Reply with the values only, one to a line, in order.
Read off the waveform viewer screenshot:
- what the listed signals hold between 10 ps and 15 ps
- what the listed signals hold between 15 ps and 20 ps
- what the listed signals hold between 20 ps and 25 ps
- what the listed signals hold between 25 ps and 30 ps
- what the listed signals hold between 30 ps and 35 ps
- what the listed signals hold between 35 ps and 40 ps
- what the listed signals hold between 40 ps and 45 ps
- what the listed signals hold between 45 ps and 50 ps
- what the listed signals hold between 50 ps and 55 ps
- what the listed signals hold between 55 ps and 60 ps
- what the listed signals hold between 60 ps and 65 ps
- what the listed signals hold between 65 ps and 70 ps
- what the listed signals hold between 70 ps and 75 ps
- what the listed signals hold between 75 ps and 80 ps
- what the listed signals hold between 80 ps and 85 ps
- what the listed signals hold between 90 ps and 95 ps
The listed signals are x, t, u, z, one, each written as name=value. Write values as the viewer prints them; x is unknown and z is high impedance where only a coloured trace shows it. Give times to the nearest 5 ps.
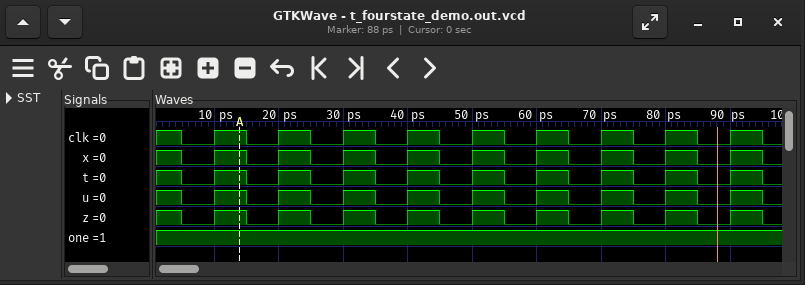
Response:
x=1, t=1, u=1, z=1, one=1
x=0, t=0, u=0, z=0, one=1
x=1, t=1, u=1, z=1, one=1
x=0, t=0, u=0, z=0, one=1
x=1, t=1, u=1, z=1, one=1
x=0, t=0, u=0, z=0, one=1
x=1, t=1, u=1, z=1, one=1
x=0, t=0, u=0, z=0, one=1
x=1, t=1, u=1, z=1, one=1
x=0, t=0, u=0, z=0, one=1
x=1, t=1, u=1, z=1, one=1
x=0, t=0, u=0, z=0, one=1
x=1, t=1, u=1, z=1, one=1
x=0, t=0, u=0, z=0, one=1
x=1, t=1, u=1, z=1, one=1
x=1, t=1, u=1, z=1, one=1
